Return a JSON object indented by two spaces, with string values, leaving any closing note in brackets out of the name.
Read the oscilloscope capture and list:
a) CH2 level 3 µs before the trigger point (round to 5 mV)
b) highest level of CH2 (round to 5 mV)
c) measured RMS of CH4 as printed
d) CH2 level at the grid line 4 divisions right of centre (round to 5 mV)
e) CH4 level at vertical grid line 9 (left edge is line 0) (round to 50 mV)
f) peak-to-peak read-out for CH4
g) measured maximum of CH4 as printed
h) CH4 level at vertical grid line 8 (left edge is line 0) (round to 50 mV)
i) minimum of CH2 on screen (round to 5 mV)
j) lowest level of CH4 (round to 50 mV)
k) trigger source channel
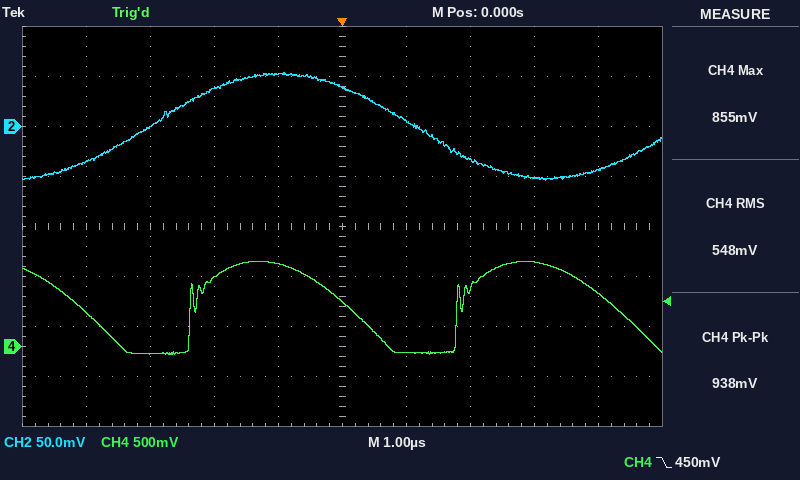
{
  "CH2 level 3 µs before the trigger point": "0 mV",
  "highest level of CH2": "55 mV",
  "measured RMS of CH4 as printed": "548 mV",
  "CH2 level at the grid line 4 divisions right of centre": "-45 mV",
  "CH4 level at vertical grid line 9 (left edge is line 0)": "550 mV",
  "peak-to-peak read-out for CH4": "938 mV",
  "measured maximum of CH4 as printed": "855 mV",
  "CH4 level at vertical grid line 8 (left edge is line 0)": "850 mV",
  "minimum of CH2 on screen": "-55 mV",
  "lowest level of CH4": "-100 mV",
  "trigger source channel": "CH4"
}
